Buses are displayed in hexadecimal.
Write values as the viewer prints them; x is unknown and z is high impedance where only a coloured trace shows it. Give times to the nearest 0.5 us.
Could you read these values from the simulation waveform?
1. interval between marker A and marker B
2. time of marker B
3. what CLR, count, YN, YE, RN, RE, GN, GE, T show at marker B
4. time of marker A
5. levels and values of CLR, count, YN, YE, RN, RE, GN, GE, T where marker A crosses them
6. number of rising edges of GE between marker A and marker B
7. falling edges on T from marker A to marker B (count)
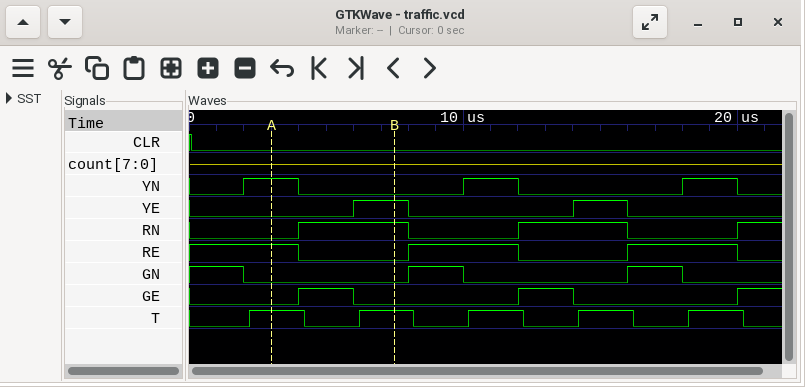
4.5 us
7.5 us
CLR=0, count=z, YN=0, YE=1, RN=1, RE=0, GN=0, GE=0, T=1
3 us
CLR=0, count=z, YN=1, YE=0, RN=0, RE=1, GN=0, GE=0, T=1
1
1
